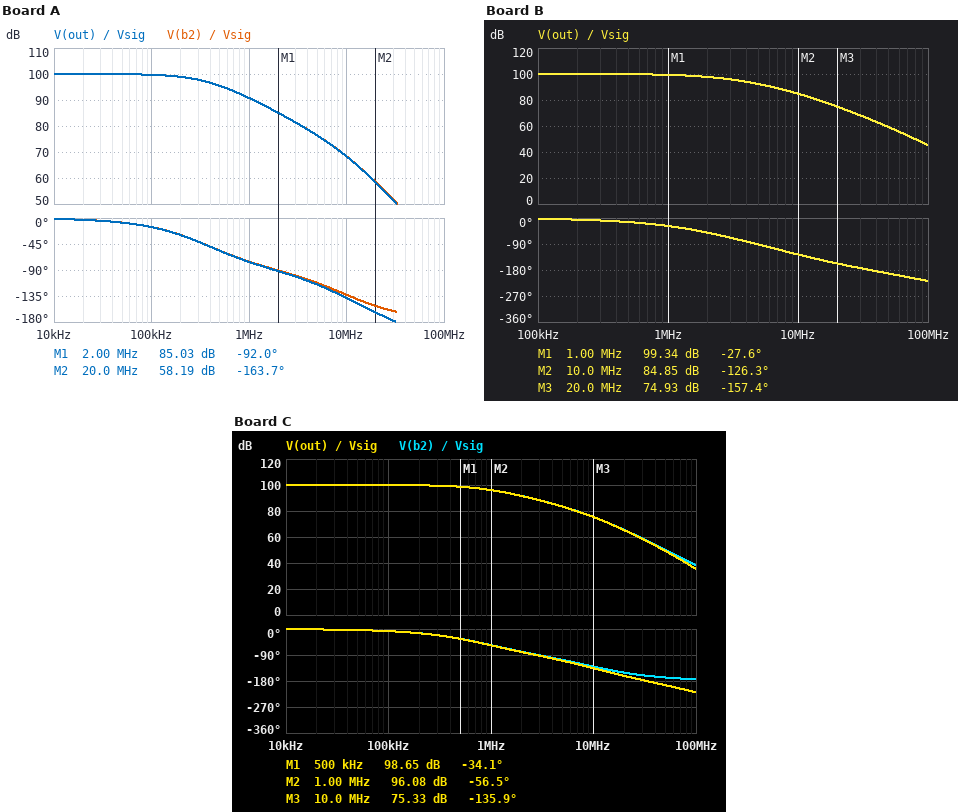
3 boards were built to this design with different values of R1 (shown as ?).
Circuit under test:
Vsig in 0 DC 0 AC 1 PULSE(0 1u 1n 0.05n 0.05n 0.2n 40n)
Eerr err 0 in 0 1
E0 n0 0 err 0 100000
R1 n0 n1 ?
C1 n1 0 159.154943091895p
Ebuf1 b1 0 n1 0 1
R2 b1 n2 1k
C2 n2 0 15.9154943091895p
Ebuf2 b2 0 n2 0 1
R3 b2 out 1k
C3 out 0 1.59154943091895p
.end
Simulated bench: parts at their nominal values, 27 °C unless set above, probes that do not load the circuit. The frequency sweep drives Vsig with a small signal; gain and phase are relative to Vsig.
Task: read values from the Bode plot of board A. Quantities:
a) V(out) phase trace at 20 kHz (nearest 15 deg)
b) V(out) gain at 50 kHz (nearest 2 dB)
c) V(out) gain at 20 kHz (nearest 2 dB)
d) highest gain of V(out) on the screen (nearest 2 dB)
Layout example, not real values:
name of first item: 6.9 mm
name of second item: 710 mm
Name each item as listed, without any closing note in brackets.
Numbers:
V(out) phase trace at 20 kHz: 0 deg
V(out) gain at 50 kHz: 100 dB
V(out) gain at 20 kHz: 100 dB
highest gain of V(out) on the screen: 100 dB
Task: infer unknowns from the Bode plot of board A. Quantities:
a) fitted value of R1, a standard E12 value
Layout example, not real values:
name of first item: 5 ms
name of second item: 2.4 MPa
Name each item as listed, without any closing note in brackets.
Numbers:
fitted value of R1, a standard E12 value: 2.7 kΩ
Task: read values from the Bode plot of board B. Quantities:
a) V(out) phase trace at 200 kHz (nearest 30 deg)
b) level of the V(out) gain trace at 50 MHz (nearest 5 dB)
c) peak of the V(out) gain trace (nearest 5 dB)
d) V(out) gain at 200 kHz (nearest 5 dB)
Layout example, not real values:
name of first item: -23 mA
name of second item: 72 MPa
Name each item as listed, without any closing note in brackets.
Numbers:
V(out) phase trace at 200 kHz: 0 deg
level of the V(out) gain trace at 50 MHz: 60 dB
peak of the V(out) gain trace: 100 dB
V(out) gain at 200 kHz: 100 dB
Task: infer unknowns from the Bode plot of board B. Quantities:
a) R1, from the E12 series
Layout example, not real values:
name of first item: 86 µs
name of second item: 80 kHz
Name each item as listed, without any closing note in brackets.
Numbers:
R1, from the E12 series: 390 Ω
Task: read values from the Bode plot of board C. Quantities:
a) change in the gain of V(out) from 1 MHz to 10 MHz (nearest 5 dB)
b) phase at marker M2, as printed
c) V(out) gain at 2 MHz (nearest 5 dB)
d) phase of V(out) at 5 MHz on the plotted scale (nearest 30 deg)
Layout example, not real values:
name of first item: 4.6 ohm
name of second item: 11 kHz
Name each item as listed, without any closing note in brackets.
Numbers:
change in the gain of V(out) from 1 MHz to 10 MHz: -20 dB
phase at marker M2, as printed: -56.5 deg
V(out) gain at 2 MHz: 90 dB
phase of V(out) at 5 MHz on the plotted scale: -120 deg
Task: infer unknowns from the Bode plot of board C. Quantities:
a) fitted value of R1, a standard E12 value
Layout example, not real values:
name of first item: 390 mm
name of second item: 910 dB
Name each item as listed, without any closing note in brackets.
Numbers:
fitted value of R1, a standard E12 value: 1.2 kΩ
